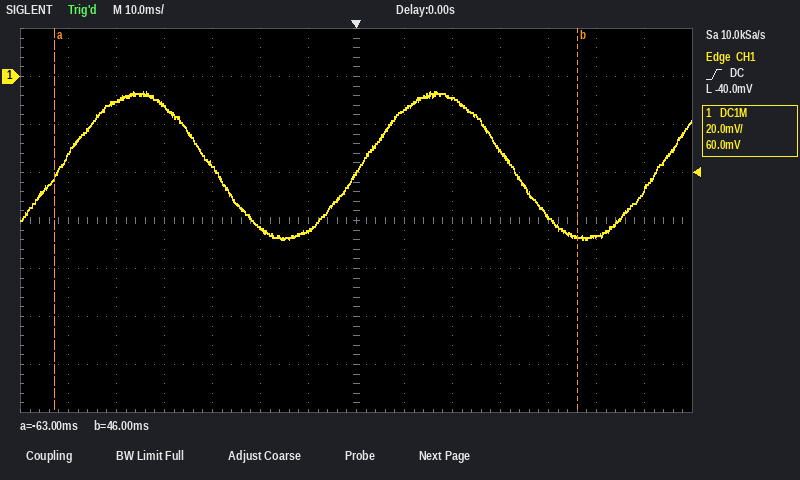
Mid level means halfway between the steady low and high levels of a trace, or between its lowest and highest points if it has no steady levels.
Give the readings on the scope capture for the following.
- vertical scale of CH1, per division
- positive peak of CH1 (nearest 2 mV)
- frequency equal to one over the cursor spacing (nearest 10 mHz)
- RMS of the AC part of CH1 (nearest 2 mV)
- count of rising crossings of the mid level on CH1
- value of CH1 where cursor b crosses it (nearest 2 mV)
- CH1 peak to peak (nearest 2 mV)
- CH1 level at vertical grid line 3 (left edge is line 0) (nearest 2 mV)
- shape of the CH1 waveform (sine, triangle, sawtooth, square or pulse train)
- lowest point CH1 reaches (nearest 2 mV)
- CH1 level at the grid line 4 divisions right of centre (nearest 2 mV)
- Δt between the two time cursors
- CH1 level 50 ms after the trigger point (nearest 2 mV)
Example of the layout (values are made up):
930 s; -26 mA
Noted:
20 mV; -6 mV; 9.17 Hz; 22 mV; 3; -66 mV; 62 mV; -12 mV; sine; -68 mV; -58 mV; 109 ms; -66 mV
